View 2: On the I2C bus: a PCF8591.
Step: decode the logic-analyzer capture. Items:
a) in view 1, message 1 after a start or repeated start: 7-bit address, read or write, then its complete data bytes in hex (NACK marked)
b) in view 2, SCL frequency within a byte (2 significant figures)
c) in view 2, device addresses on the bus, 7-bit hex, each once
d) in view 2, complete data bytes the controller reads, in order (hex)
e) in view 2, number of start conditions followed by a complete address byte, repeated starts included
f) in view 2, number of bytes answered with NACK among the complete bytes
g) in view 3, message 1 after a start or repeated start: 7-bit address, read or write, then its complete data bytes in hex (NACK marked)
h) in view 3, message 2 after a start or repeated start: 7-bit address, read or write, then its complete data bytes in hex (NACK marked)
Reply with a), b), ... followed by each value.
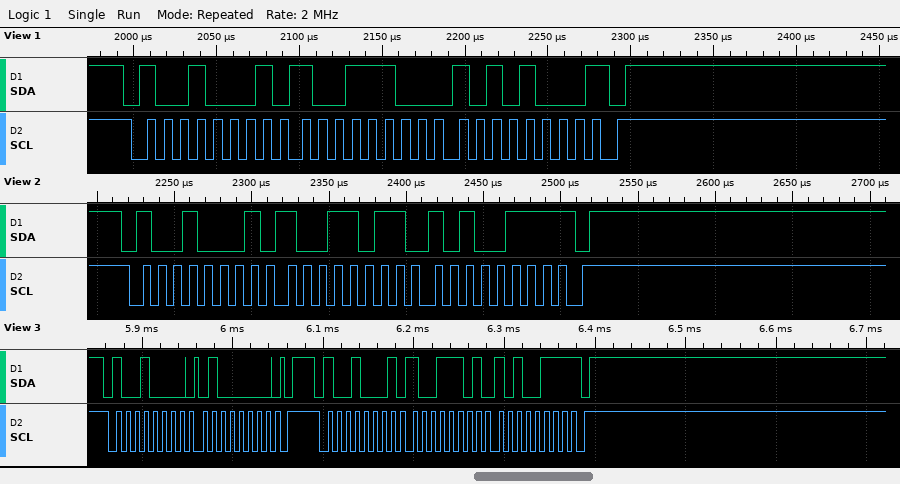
a) 0x48 read: 9C A8 NACK
b) 100 kHz
c) 0x48
d) 9B A7
e) 1
f) 1
g) 0x48 write: 40
h) 0x48 read: 9D A7 NACK
